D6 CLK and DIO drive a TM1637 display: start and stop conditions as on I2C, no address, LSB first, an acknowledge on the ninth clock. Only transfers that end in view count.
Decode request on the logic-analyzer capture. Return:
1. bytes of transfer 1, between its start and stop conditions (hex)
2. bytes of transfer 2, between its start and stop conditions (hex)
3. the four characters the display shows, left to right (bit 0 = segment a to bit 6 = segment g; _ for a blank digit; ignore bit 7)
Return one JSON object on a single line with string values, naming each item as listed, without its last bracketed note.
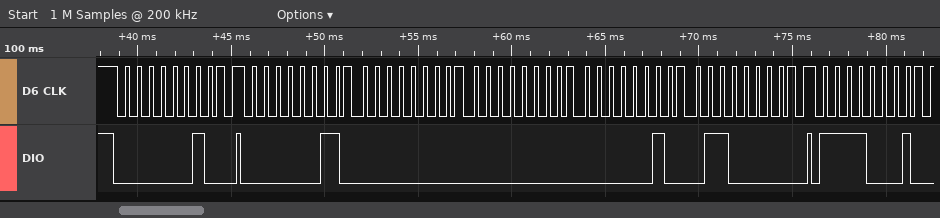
{"bytes of transfer 1, between its start and stop conditions": "40", "bytes of transfer 2, between its start and stop conditions": "C0 00 00 40 06", "the four characters the display shows, left to right": "__-1"}
